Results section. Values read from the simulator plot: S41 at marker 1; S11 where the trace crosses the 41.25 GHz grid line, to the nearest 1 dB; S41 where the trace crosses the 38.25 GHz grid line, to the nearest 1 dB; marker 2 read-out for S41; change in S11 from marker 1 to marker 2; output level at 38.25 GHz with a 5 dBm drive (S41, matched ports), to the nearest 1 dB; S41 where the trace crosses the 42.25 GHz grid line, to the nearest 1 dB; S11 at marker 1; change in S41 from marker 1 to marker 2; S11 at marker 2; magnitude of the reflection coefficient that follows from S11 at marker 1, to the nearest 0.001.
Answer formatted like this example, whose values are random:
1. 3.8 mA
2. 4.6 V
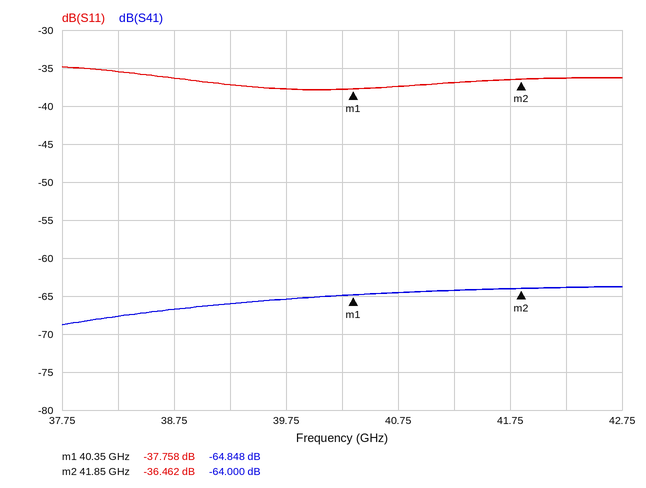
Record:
1. -64.848 dB
2. -37 dB
3. -68 dB
4. -64.000 dB
5. 1.296 dB
6. -63 dBm
7. -64 dB
8. -37.758 dB
9. 0.848 dB
10. -36.462 dB
11. 0.013
